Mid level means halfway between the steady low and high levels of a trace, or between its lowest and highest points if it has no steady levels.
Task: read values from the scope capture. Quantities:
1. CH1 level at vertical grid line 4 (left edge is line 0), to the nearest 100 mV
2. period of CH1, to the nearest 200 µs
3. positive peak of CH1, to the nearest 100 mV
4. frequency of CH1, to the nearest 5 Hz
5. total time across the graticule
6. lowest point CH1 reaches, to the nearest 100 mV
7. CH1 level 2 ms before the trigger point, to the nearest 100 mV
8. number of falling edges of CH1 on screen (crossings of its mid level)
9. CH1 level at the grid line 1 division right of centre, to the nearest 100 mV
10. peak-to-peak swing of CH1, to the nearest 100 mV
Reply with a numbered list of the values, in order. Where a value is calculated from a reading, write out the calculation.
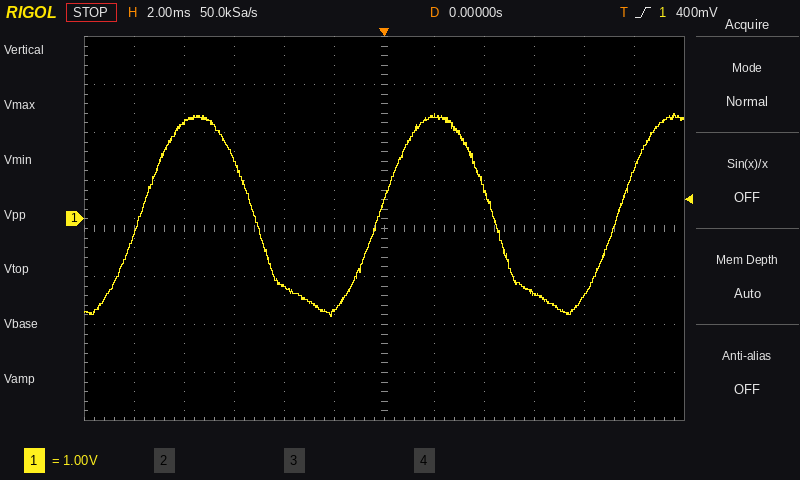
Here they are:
1. -1.4 V
2. 9.6 ms
3. 2.2 V
4. 1 / 9.6 ms ≈ 104 Hz, so 105 Hz to the nearest 5 Hz
5. 24 ms
6. -2.0 V
7. -1.9 V
8. 2
9. 2.2 V
10. 2.2 V − (-2.0 V) = 4.2 V
